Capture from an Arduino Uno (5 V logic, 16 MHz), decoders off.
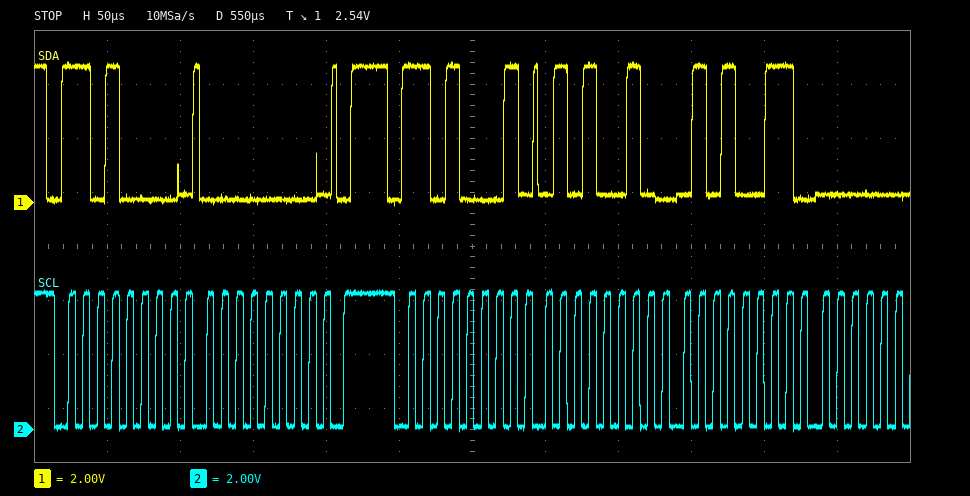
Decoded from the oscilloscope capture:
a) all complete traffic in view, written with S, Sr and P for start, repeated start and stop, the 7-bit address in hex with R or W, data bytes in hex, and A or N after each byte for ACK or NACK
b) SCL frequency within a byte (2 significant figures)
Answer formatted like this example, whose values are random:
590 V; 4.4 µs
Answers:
S 68W A 00 A P S 68R A 52 A 53 A; 100 kHz
